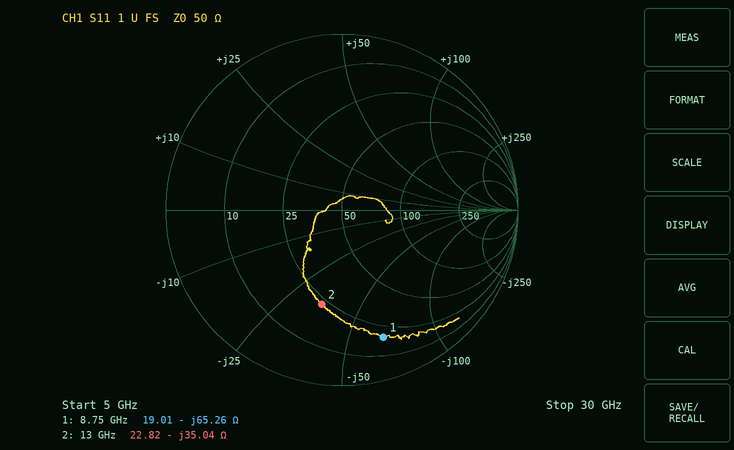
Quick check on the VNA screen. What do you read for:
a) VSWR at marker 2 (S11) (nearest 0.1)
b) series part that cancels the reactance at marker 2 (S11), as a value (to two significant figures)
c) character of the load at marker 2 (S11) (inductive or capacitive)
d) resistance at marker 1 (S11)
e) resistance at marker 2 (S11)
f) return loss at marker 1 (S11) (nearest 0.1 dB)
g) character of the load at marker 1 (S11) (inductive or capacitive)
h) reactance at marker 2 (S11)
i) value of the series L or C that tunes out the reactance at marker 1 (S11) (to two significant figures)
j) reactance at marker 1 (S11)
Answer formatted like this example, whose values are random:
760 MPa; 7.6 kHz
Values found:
3.4; 430 pH; capacitive; 19.01 Ω; 22.82 Ω; 2.4 dB; capacitive; -35.04 Ω; 1.2 nH; -65.26 Ω
